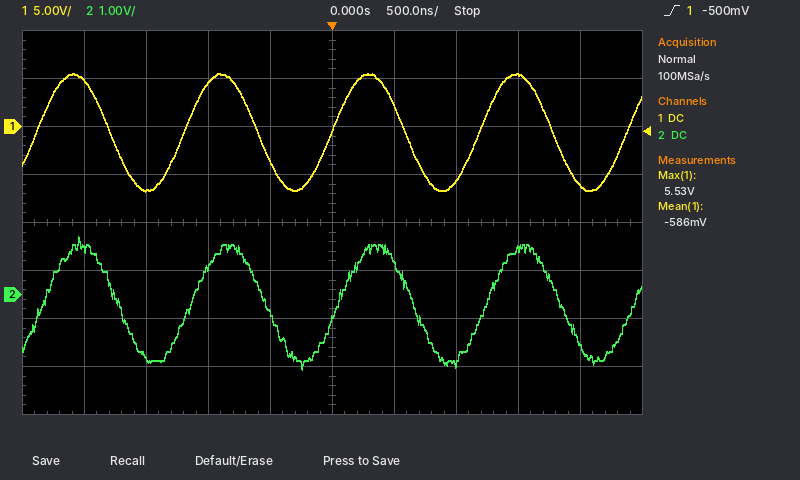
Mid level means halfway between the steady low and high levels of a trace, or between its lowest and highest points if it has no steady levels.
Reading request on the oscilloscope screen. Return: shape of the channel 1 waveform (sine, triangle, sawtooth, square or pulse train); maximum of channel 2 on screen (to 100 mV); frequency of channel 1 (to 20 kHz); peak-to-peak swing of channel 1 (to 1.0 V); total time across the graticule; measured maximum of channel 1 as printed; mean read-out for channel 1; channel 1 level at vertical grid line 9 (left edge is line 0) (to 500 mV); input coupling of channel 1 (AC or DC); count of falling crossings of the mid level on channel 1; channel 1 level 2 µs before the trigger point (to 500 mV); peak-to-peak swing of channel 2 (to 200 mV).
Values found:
sine
1.2 V
840 kHz
12.0 V
5 µs
5.53 V
-586 mV
-6.0 V
DC
4
5.0 V
2.8 V
